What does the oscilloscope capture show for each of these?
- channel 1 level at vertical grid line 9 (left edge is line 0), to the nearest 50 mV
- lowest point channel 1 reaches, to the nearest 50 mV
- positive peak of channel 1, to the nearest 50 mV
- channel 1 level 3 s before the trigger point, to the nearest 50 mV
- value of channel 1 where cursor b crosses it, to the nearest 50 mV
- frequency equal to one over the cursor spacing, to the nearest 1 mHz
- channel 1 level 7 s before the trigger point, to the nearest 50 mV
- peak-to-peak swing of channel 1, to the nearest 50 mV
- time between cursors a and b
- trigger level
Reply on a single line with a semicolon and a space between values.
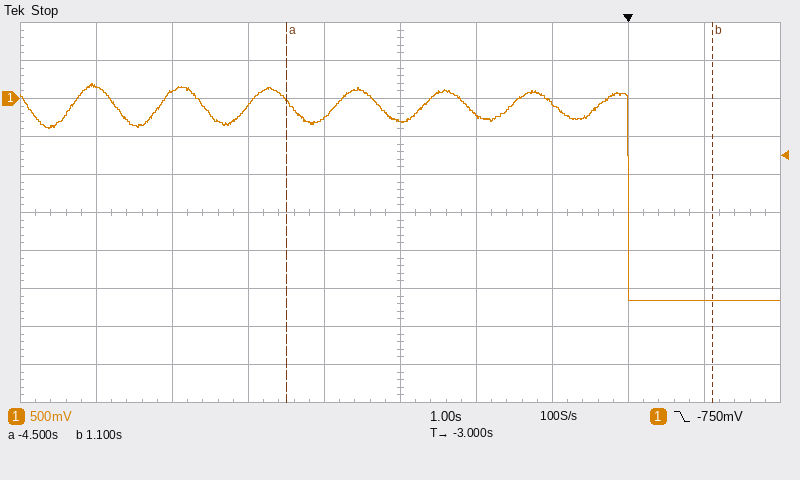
-2.65 V; -2.65 V; 200 mV; -300 mV; -2.65 V; 179 mHz; 150 mV; 2.85 V; 5.6 s; -750 mV
